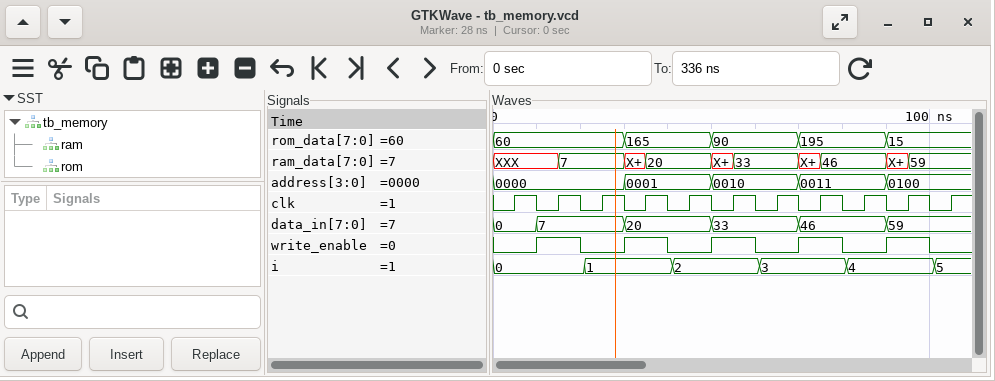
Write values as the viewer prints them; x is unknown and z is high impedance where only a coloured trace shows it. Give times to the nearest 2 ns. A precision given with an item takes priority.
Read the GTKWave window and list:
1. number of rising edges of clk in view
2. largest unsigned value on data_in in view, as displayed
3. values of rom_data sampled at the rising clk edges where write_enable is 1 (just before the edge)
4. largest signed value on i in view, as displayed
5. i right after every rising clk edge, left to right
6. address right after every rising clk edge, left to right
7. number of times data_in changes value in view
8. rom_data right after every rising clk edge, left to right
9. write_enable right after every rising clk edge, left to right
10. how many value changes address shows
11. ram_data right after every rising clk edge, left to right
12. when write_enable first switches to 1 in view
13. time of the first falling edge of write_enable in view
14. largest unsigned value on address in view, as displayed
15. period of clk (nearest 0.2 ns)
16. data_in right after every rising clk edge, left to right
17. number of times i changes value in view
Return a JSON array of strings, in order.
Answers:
["11", "59", "60, 165, 90, 195, 15", "5", "0, 0, 1, 1, 2, 2, 3, 3, 4, 4, 5", "0000, 0000, 0000, 0001, 0001, 0010, 0010, 0011, 0011, 0100, 0100", "5", "60, 60, 60, 165, 165, 90, 90, 195, 195, 15, 15", "0 1 0 1 0 1 0 1 0 1 0", "4", "XXX, 7, 7, 20, 20, 33, 33, 46, 46, 59, 59", "10 ns", "20 ns", "0100", "10 ns", "0, 7, 7, 20, 20, 33, 33, 46, 46, 59, 59", "5"]
